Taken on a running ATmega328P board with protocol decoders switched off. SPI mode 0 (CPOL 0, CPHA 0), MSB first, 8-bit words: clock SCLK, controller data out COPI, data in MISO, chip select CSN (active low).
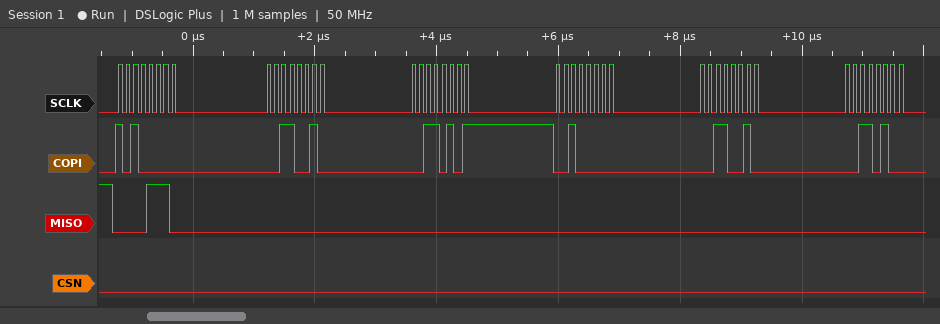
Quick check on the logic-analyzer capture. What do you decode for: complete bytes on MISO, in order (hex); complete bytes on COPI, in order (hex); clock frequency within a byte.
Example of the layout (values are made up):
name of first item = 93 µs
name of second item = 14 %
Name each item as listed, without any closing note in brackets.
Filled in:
complete bytes on MISO, in order = 0x0E 0x00 0x00 0x00 0x00 0x00
complete bytes on COPI, in order = 0xA0 0x32 0x35 0x20 0x32 0x34
clock frequency within a byte = 8 MHz
